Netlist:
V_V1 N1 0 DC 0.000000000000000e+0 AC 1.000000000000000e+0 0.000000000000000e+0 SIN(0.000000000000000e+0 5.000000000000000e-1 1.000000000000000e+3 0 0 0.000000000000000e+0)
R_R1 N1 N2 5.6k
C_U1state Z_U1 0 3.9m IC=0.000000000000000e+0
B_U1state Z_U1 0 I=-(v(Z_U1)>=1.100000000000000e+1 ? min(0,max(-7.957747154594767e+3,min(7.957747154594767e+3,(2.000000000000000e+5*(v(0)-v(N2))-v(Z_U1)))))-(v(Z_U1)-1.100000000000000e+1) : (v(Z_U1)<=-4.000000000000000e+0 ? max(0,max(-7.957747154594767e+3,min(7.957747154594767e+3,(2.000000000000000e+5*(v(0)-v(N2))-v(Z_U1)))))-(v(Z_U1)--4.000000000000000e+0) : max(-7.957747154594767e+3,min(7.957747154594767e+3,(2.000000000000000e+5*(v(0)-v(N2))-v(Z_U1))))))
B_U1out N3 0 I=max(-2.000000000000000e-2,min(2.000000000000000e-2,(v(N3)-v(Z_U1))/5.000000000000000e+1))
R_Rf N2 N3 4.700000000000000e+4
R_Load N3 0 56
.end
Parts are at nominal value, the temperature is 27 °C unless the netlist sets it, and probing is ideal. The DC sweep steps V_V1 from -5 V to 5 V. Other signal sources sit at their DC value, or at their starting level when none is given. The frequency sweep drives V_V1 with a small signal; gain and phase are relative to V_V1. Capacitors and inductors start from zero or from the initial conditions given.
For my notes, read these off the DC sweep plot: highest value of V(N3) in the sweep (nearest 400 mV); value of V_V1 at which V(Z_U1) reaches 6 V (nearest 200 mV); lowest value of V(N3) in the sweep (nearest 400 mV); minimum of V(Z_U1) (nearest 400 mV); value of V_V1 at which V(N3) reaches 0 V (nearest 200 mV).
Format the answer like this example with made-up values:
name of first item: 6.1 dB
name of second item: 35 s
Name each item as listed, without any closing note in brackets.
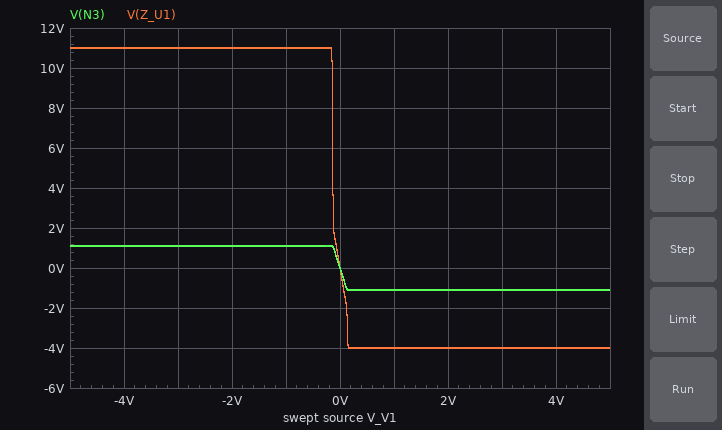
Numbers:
highest value of V(N3) in the sweep: 1.2 V
value of V_V1 at which V(Z_U1) reaches 6 V: -200 mV
lowest value of V(N3) in the sweep: -1.2 V
minimum of V(Z_U1): -4.0 V
value of V_V1 at which V(N3) reaches 0 V: 0 V
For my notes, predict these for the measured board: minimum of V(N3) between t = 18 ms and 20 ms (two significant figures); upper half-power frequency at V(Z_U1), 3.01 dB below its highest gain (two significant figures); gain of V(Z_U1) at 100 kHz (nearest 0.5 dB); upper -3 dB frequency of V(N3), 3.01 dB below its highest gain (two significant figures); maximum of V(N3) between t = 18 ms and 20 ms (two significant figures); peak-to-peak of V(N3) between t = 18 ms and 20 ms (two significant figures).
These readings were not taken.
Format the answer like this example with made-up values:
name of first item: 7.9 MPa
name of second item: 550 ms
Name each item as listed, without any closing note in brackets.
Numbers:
minimum of V(N3) between t = 18 ms and 20 ms: -1.1 V
upper half-power frequency at V(Z_U1), 3.01 dB below its highest gain: 460 kHz
gain of V(Z_U1) at 100 kHz: 24.0 dB
upper -3 dB frequency of V(N3), 3.01 dB below its highest gain: 460 kHz
maximum of V(N3) between t = 18 ms and 20 ms: 1.1 V
peak-to-peak of V(N3) between t = 18 ms and 20 ms: 2.2 V
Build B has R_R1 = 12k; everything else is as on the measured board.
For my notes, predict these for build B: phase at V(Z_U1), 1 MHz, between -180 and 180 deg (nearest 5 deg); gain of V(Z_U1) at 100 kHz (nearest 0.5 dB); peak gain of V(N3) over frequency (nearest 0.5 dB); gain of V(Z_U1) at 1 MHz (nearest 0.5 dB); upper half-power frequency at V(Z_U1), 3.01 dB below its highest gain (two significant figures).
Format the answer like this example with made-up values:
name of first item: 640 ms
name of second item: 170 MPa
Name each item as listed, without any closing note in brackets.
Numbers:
phase at V(Z_U1), 1 MHz, between -180 and 180 deg: 130 deg
gain of V(Z_U1) at 100 kHz: 17.5 dB
peak gain of V(N3) over frequency: 12.0 dB
gain of V(Z_U1) at 1 MHz: 14.0 dB
upper half-power frequency at V(Z_U1), 3.01 dB below its highest gain: 880 kHz
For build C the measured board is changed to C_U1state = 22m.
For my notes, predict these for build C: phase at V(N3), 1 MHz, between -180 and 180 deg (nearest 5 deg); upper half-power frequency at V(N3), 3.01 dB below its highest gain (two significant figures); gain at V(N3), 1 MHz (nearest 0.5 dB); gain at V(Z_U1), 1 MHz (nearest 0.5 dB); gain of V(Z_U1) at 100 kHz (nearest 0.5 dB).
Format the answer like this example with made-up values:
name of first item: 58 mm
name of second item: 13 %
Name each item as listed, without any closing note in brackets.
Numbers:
phase at V(N3), 1 MHz, between -180 and 180 deg: 95 deg
upper half-power frequency at V(N3), 3.01 dB below its highest gain: 81 kHz
gain at V(N3), 1 MHz: -3.5 dB
gain at V(Z_U1), 1 MHz: 2.0 dB
gain of V(Z_U1) at 100 kHz: 20.0 dB
